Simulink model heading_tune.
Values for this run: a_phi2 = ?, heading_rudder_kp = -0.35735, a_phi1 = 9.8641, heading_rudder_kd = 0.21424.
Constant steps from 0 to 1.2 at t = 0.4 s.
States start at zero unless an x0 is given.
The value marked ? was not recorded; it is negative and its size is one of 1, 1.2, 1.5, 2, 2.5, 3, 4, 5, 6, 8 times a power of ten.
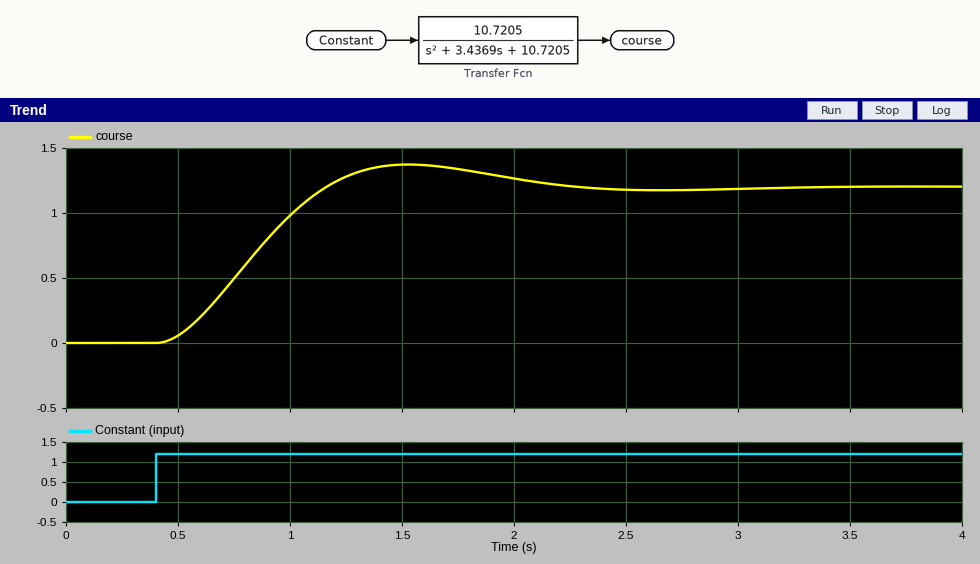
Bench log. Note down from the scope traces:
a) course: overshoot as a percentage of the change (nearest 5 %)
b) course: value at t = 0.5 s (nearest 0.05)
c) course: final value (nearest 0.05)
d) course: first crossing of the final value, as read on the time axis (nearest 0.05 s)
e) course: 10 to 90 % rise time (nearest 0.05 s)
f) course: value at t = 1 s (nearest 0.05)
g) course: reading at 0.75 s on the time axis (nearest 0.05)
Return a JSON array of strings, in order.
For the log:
["15 %", "0.05", "1.20", "1.15 s", "0.50 s", "1.00", "0.50"]
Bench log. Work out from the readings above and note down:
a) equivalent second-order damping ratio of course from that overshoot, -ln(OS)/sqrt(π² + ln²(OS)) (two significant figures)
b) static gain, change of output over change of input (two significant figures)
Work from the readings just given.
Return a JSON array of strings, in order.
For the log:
["0.52", "1.0"]
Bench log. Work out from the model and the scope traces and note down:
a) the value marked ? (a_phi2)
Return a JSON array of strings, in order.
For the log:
["-30"]
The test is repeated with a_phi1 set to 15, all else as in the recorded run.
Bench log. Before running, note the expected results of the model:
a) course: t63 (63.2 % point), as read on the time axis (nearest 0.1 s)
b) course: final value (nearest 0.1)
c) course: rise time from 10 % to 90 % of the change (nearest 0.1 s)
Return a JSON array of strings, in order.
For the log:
["1.2 s", "1.2", "1.5 s"]
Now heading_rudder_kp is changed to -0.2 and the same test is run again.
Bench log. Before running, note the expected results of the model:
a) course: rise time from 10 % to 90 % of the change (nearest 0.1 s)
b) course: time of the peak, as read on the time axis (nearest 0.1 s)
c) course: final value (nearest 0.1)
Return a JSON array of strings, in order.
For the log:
["0.9 s", "2.2 s", "1.2"]
